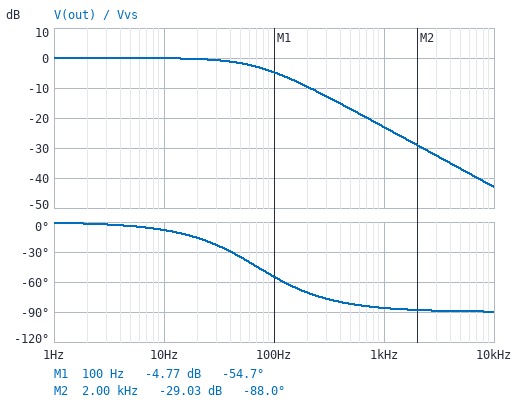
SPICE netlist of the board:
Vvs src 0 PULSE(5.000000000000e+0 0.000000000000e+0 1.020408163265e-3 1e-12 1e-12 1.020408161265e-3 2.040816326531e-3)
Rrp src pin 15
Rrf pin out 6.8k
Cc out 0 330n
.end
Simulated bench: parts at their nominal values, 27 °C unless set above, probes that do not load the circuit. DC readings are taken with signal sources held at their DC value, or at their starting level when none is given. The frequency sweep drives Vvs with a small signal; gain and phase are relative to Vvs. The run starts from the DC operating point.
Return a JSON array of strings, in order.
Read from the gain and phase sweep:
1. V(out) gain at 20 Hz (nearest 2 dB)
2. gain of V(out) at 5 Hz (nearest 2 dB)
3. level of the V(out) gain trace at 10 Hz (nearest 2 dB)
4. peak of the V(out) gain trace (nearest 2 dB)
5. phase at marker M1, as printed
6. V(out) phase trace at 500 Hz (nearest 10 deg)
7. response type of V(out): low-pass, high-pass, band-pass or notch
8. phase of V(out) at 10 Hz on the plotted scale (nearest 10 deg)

["0 dB", "0 dB", "0 dB", "0 dB", "-54.7 deg", "-80 deg", "low-pass", "-10 deg"]
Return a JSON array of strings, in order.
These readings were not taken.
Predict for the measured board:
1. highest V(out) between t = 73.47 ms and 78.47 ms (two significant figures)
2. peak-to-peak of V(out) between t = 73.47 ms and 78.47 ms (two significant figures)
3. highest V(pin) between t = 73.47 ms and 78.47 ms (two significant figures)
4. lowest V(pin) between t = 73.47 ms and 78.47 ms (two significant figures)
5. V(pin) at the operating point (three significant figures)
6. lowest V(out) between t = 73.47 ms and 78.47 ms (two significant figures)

["3.1 V", "1.1 V", "5.0 V", "4.3 mV", "5.00 V", "1.9 V"]
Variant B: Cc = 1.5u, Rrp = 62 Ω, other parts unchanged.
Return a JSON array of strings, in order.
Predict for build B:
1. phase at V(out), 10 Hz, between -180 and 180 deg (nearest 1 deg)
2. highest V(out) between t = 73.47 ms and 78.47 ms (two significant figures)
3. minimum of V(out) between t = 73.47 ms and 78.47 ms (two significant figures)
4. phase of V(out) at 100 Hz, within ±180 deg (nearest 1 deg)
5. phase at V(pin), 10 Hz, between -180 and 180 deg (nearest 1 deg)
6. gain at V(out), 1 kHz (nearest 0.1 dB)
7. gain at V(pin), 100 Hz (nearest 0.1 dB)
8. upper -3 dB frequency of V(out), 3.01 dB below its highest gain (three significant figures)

["-33 deg", "2.6 V", "2.4 V", "-81 deg", "0 deg", "-36.2 dB", "-0.1 dB", "15.5 Hz"]
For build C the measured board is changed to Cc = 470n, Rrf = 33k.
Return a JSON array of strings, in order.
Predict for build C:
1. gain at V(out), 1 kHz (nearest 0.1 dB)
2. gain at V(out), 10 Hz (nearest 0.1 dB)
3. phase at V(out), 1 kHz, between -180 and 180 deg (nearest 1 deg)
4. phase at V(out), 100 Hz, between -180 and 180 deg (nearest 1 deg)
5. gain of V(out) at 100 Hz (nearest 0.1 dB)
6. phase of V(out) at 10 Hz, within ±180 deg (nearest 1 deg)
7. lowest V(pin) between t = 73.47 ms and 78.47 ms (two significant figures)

["-39.8 dB", "-2.9 dB", "-89 deg", "-84 deg", "-19.8 dB", "-44 deg", "1.1 mV"]
